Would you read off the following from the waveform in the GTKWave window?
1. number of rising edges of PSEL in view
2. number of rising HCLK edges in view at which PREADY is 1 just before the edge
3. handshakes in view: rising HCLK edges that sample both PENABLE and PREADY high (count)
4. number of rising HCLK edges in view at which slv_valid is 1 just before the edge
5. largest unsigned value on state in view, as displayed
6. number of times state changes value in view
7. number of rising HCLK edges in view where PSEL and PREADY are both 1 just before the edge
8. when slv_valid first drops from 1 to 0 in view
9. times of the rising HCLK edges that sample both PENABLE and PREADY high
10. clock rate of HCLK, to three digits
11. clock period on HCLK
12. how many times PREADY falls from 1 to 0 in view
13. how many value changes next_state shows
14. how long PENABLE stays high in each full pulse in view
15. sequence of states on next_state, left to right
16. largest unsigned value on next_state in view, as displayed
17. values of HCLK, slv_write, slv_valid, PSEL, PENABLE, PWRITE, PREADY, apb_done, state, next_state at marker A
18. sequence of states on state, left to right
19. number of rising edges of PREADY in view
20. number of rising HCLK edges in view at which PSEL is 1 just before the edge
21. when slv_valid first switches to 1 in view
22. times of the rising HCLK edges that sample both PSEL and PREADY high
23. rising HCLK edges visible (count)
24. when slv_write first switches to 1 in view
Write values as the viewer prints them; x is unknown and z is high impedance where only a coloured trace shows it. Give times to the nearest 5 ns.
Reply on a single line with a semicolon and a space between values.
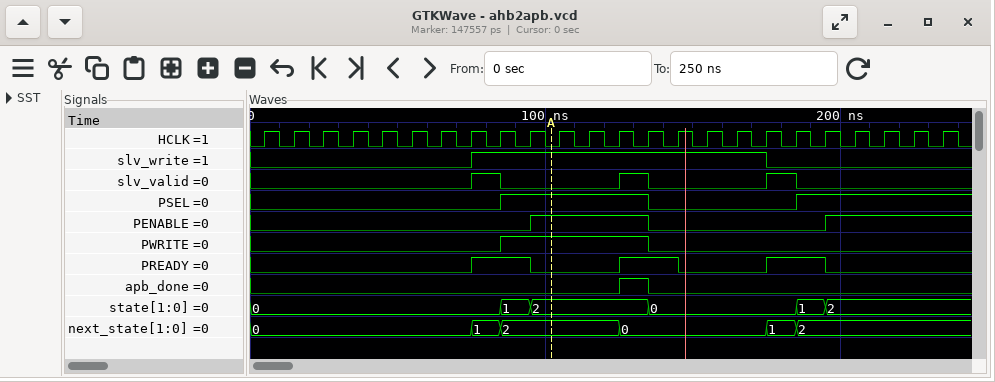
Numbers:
2; 6; 1; 3; 2; 5; 3; 85 ns; 135 ns; 100 MHz; 10 ns; 3; 5; 40 ns; 0, 1, 2, 0, 1, 2; 2; HCLK=0, slv_write=1, slv_valid=0, PSEL=1, PENABLE=1, PWRITE=1, PREADY=0, apb_done=0, state=2, next_state=2; 0, 1, 2, 0, 1, 2; 3; 10; 75 ns; 95 ns, 135 ns, 195 ns; 24; 75 ns
